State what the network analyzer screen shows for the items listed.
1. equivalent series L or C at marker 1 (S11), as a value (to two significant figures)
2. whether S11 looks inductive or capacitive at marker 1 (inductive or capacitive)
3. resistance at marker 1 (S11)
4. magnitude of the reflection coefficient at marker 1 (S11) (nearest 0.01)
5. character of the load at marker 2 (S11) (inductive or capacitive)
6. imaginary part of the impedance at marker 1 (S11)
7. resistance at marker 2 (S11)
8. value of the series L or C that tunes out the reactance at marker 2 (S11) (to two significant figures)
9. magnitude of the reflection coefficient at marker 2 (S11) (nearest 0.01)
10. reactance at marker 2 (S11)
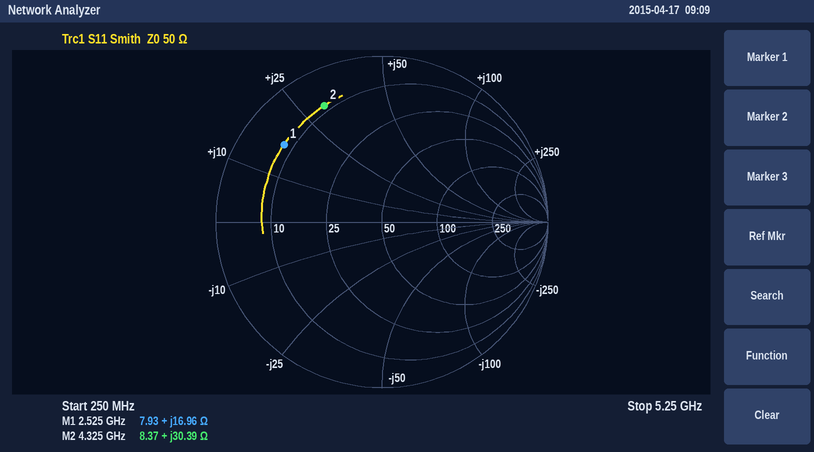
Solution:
1.1 nH
inductive
7.93 Ω
0.75
inductive
+16.96 Ω
8.37 Ω
1.2 pF
0.78
+30.39 Ω
